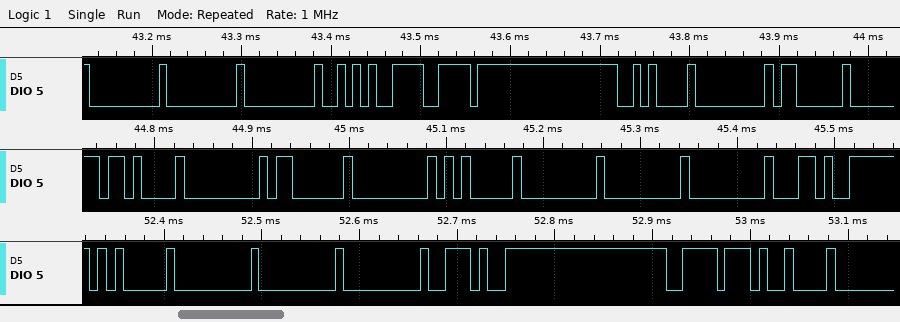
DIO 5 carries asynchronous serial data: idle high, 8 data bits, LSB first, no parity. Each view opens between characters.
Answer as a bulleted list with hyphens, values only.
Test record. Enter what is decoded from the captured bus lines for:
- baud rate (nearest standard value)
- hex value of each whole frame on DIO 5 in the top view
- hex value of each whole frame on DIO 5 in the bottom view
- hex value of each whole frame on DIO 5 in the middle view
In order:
- 115200 baud
- 00, 00, 00, 2A, DE, 0A, 00, 03
- 05, 00, 00, 00, 2E, DE, 09
- 0B, 00, 03, 00, 05, 00, 00, 00, 2C
